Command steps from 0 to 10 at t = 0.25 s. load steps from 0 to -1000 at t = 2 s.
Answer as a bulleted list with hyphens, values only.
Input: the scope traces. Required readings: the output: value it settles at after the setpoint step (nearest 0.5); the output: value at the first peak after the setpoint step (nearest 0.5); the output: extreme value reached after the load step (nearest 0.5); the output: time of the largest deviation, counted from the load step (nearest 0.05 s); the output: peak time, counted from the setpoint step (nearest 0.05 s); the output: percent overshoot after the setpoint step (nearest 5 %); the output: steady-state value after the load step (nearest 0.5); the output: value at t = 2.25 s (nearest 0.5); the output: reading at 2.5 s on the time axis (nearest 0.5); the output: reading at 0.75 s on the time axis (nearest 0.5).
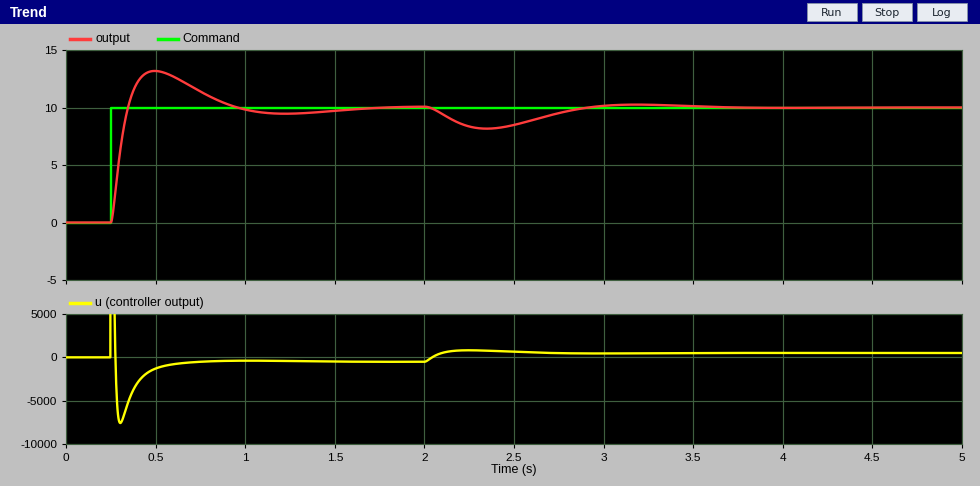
- 10.0
- 13.0
- 8.0
- 0.35 s
- 0.25 s
- 30 %
- 10.0
- 8.5
- 8.5
- 11.5
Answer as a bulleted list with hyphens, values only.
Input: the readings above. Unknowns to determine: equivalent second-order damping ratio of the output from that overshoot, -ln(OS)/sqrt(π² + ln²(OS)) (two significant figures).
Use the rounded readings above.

- 0.36
